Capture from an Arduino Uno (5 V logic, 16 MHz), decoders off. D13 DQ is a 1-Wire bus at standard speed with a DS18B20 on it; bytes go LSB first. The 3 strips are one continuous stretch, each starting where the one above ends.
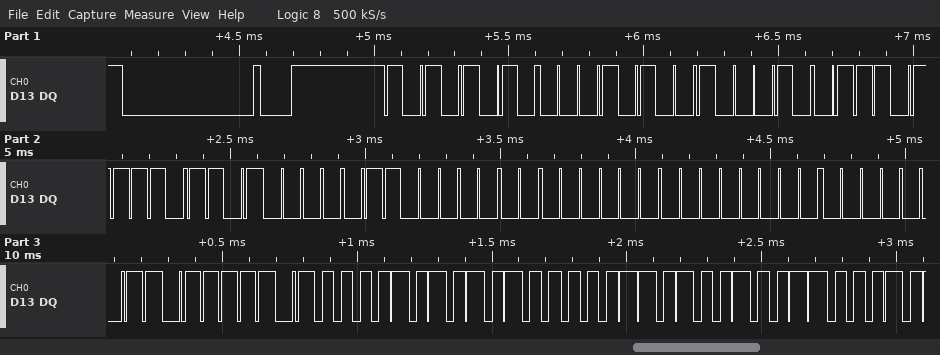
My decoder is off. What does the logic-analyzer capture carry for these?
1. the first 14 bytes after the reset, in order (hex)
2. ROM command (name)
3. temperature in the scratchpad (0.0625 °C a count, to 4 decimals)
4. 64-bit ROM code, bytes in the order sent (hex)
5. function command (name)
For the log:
55 28 91 7B 0B 06 00 00 C0 BE 50 05 4B 46
Match ROM
85.0000 °C
28 91 7B 0B 06 00 00 C0
Read Scratchpad
